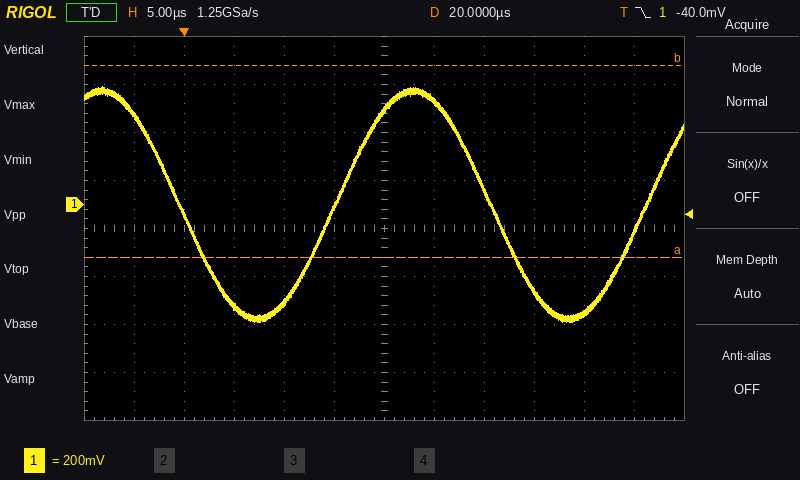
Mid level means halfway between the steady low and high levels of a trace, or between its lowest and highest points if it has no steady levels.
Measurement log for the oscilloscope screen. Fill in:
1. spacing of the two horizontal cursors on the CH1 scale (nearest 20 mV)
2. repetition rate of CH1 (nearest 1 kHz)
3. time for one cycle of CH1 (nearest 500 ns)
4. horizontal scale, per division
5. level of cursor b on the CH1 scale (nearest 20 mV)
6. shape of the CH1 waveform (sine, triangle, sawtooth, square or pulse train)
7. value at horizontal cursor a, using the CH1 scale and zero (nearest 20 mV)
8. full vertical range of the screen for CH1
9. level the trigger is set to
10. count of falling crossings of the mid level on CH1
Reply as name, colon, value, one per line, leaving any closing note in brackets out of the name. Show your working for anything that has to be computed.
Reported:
spacing of the two horizontal cursors on the CH1 scale: 800 mV
repetition rate of CH1: 1 / 31.0 µs ≈ 32 kHz
time for one cycle of CH1: 31.0 µs
horizontal scale, per division: 5 µs
level of cursor b on the CH1 scale: 580 mV
shape of the CH1 waveform: sine
value at horizontal cursor a, using the CH1 scale and zero: -220 mV
full vertical range of the screen for CH1: 1.6 V
level the trigger is set to: -40.0 mV
count of falling crossings of the mid level on CH1: 2
